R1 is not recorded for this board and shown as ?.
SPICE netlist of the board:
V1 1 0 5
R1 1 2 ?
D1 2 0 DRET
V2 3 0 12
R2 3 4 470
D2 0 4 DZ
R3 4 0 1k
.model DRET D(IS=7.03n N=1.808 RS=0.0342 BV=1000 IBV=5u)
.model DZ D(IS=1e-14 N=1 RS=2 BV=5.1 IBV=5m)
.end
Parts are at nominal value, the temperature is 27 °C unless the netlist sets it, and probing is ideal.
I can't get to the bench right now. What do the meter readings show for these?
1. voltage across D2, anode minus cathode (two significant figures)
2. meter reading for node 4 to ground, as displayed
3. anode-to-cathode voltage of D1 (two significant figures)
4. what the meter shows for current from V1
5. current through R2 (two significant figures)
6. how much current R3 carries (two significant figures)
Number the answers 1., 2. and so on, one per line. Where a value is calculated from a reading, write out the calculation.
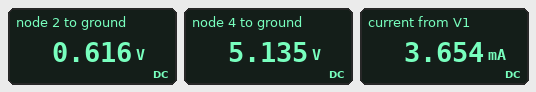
1. 0 V - 5.135 V = -5.1 V
2. 5.135 V
3. 616 mV = 620 mV
4. 3.654 mA
5. (12 V - 5.135 V) / 470 Ω = 15 mA
6. (5.135 V) / 1 kΩ = 5.1 mA
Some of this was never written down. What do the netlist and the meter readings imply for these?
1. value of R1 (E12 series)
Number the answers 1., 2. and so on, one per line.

1. 1.2 kΩ
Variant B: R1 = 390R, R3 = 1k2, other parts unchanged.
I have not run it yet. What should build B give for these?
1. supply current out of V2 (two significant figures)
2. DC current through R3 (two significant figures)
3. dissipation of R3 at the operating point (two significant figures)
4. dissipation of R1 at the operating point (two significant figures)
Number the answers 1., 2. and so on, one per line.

1. 15 mA
2. 4.3 mA
3. 22 mW
4. 48 mW
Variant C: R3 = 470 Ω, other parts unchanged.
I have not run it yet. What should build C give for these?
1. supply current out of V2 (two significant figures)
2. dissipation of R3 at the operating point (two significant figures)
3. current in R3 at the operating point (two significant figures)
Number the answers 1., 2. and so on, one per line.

1. 15 mA
2. 55 mW
3. 11 mA
